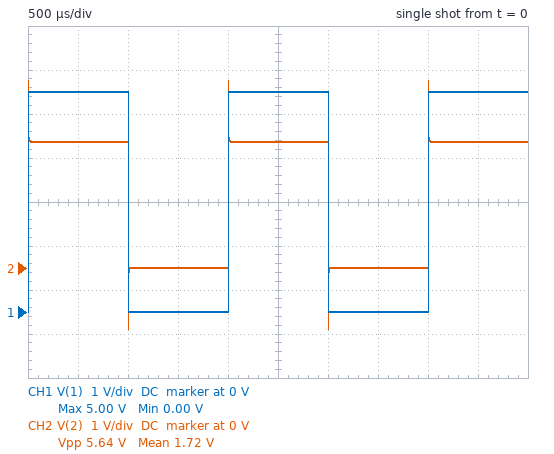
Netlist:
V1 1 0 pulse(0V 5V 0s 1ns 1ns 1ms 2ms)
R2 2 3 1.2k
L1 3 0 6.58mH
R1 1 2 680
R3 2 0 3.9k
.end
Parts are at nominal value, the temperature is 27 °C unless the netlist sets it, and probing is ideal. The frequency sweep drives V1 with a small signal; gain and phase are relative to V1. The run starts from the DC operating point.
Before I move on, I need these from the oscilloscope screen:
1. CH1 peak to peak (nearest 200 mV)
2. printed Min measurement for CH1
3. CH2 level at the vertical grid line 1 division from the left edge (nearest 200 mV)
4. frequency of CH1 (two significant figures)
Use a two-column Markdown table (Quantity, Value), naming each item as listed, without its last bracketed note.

| Quantity | Value |
|---|---|
| CH1 peak to peak | 5.0 V |
| printed Min measurement for CH1 | 0.00 V |
| CH2 level at the vertical grid line 1 division from the left edge | 2.8 V |
| frequency of CH1 | 500 Hz |
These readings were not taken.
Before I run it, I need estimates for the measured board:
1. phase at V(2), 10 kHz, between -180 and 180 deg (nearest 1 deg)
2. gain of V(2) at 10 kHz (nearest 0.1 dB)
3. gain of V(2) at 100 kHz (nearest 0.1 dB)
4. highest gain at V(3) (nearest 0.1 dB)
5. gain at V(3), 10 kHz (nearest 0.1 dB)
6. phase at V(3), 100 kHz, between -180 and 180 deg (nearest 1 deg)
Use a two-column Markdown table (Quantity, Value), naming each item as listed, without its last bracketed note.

| Quantity | Value |
|---|---|
| phase at V(2), 10 kHz, between -180 and 180 deg | 6 deg |
| gain of V(2) at 10 kHz | -4.6 dB |
| gain of V(2) at 100 kHz | -1.8 dB |
| highest gain at V(3) | -1.4 dB |
| gain at V(3), 10 kHz | -14.3 dB |
| phase at V(3), 100 kHz, between -180 and 180 deg | 23 deg |
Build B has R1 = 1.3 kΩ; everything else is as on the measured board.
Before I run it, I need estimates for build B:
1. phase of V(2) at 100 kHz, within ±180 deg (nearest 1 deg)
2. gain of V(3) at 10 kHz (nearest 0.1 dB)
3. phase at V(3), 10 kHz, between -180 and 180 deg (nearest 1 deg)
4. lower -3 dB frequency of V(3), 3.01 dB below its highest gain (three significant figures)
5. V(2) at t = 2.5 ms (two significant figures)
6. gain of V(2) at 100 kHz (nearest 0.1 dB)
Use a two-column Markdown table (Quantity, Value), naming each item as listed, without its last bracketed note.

| Quantity | Value |
|---|---|
| phase of V(2) at 100 kHz, within ±180 deg | 12 deg |
| gain of V(3) at 10 kHz | -17.1 dB |
| phase at V(3), 10 kHz, between -180 and 180 deg | 79 deg |
| lower -3 dB frequency of V(3), 3.01 dB below its highest gain | 52.6 kHz |
| V(2) at t = 2.5 ms | 2.1 V |
| gain of V(2) at 100 kHz | -3.2 dB |
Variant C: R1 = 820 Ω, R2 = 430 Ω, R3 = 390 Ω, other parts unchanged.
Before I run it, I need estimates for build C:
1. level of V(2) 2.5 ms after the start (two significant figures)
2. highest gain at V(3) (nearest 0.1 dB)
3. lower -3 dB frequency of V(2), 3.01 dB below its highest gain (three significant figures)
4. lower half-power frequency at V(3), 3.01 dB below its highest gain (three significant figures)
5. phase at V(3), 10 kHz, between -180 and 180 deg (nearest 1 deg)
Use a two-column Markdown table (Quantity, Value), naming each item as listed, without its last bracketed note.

| Quantity | Value |
|---|---|
| level of V(2) 2.5 ms after the start | 1.0 V |
| highest gain at V(3) | -9.8 dB |
| lower -3 dB frequency of V(2), 3.01 dB below its highest gain | 8.10 kHz |
| lower half-power frequency at V(3), 3.01 dB below its highest gain | 16.8 kHz |
| phase at V(3), 10 kHz, between -180 and 180 deg | 59 deg |
